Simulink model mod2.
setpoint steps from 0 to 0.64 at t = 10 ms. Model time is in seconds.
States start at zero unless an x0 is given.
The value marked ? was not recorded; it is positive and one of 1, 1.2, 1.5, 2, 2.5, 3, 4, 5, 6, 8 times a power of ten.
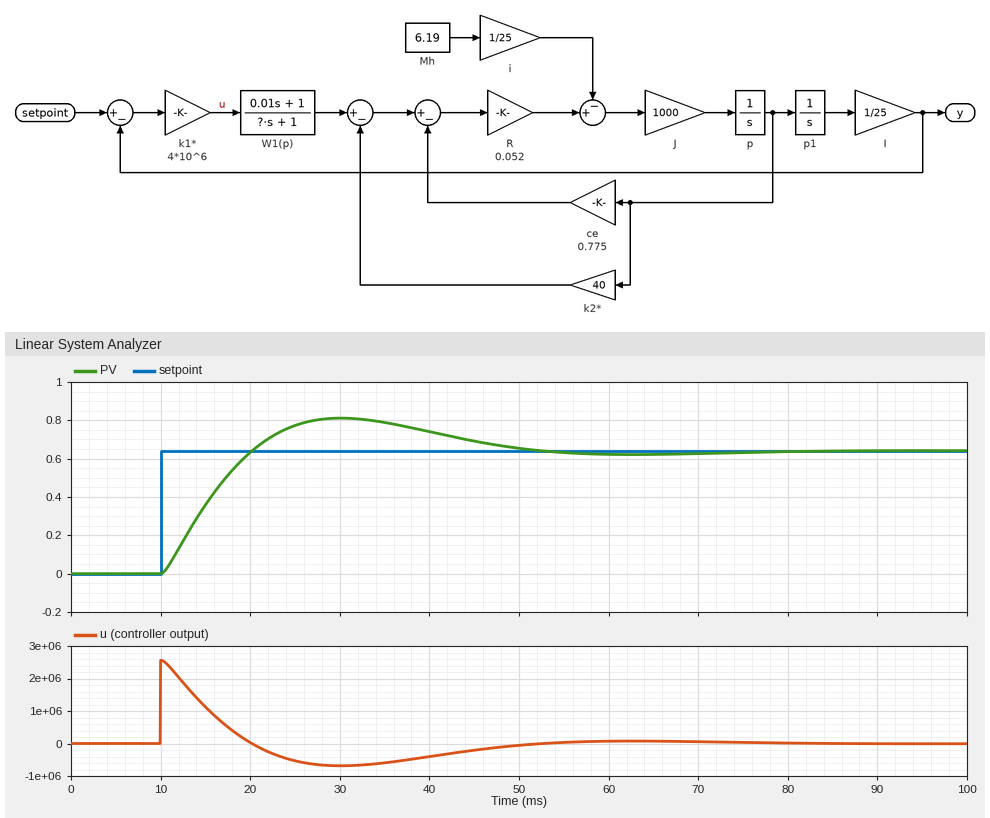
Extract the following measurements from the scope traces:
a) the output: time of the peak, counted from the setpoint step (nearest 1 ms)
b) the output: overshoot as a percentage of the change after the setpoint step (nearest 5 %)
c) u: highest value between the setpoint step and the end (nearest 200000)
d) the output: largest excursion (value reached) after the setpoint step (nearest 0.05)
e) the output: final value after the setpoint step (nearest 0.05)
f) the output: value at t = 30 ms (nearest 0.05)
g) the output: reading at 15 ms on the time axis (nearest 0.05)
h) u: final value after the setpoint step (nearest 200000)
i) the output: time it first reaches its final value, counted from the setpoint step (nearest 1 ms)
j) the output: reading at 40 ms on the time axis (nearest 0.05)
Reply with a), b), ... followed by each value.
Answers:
a) 20 ms
b) 25 %
c) 2600000
d) 0.80
e) 0.65
f) 0.80
g) 0.35
h) 0
i) 10 ms
j) 0.75
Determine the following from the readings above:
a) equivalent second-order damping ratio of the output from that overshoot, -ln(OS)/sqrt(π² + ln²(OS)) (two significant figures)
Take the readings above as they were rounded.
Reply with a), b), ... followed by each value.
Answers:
a) 0.40
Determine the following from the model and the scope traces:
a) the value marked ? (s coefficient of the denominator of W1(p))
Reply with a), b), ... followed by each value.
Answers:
a) 0.3
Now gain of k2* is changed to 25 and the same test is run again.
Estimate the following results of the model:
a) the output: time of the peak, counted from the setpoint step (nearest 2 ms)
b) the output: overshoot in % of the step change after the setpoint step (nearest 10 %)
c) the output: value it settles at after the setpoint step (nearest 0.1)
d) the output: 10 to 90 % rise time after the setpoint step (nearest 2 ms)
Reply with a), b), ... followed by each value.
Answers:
a) 14 ms
b) 20 %
c) 0.6
d) 6 ms
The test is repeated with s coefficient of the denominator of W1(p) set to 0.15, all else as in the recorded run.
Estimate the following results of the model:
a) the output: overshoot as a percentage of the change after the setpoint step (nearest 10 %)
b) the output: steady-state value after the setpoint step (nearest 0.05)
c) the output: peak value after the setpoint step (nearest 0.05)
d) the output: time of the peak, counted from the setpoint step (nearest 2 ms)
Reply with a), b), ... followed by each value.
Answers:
a) 20 %
b) 0.65
c) 0.75
d) 12 ms
